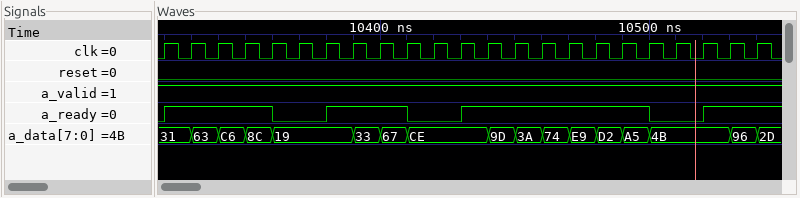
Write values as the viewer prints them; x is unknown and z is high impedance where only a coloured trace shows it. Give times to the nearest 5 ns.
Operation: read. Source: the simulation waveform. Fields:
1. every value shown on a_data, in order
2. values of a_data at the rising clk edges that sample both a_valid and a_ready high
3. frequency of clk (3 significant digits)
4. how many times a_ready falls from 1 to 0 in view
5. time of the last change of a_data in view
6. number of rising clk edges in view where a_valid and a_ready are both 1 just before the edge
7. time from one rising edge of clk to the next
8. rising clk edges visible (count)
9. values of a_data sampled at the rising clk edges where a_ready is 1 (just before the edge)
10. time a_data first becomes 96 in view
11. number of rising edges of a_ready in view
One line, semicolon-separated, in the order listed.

31, 63, C6, 8C, 19, 33, 67, CE, 9D, 3A, 74, E9, D2, A5, 4B, 96, 2D; 31, 63, C6, 8C, 19, 33, 67, CE, 9D, 3A, 74, E9, D2, A5, 4B, 96; 100 MHz; 3; 10540 ns; 16; 10 ns; 23; 31, 63, C6, 8C, 19, 33, 67, CE, 9D, 3A, 74, E9, D2, A5, 4B, 96; 10530 ns; 4
